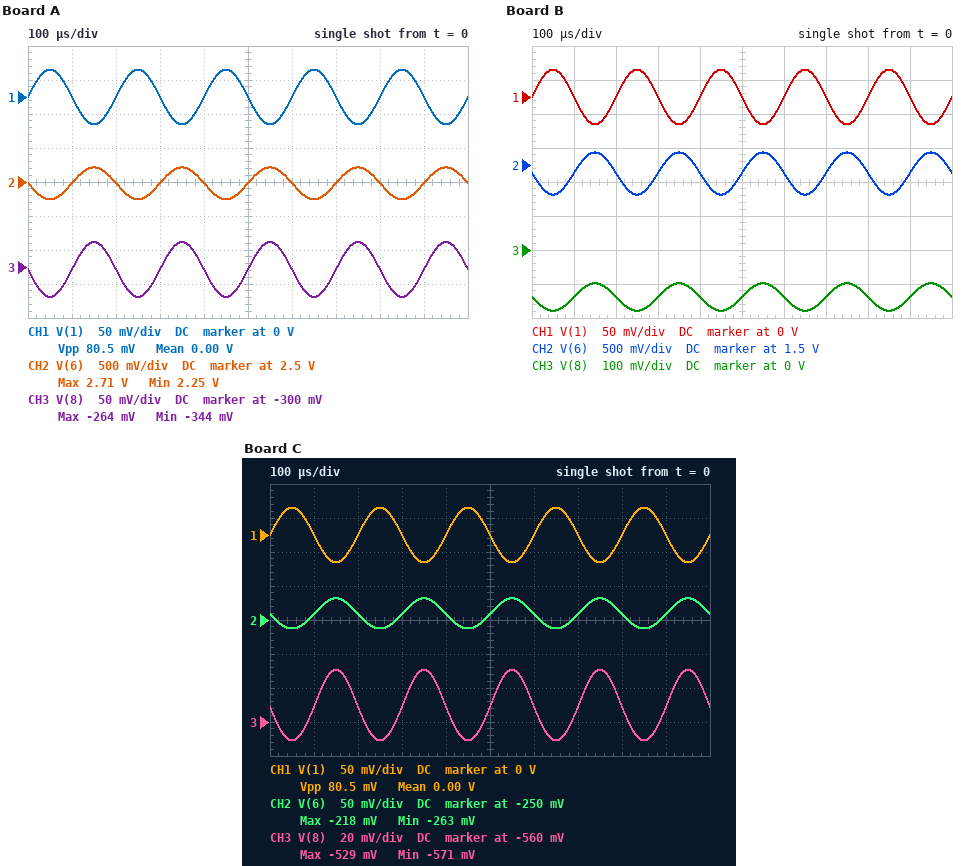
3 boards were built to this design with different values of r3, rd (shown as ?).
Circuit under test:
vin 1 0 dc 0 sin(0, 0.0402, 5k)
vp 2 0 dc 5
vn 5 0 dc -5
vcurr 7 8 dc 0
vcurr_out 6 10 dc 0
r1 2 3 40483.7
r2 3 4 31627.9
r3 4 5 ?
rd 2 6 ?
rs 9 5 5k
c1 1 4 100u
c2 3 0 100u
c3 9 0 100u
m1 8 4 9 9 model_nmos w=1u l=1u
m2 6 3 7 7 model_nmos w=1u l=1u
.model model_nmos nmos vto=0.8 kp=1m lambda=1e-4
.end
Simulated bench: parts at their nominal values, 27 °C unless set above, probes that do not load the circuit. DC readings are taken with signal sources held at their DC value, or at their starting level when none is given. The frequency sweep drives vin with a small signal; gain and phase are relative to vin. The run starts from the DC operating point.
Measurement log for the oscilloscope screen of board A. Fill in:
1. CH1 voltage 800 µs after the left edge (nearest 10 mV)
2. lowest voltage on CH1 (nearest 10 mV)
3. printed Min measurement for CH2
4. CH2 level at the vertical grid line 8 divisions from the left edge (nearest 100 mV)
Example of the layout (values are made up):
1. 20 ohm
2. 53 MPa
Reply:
1. 0 V
2. -40 mV
3. 2.25 V
4. 2.5 V
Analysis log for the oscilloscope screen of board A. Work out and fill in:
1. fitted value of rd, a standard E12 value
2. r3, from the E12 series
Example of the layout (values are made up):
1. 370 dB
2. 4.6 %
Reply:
1. 6.8 kΩ
2. 39 kΩ
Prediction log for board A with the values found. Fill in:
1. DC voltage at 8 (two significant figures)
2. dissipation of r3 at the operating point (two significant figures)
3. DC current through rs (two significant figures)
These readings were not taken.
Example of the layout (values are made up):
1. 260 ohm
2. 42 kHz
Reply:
1. -300 mV
2. 320 µW
3. 370 µA
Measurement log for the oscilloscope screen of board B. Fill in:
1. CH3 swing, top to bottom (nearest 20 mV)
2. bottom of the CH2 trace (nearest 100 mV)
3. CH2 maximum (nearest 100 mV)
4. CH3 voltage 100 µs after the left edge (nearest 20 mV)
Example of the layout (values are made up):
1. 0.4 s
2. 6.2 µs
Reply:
1. 80 mV
2. 1.1 V
3. 1.7 V
4. -140 mV
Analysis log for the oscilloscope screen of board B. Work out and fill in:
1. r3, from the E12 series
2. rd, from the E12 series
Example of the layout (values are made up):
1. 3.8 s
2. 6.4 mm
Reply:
1. 47 kΩ
2. 8.2 kΩ
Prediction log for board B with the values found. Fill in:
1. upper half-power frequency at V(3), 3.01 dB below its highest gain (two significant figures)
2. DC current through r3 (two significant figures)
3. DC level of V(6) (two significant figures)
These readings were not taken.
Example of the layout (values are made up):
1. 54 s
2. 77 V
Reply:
1. 200 mHz
2. 84 µA
3. 1.4 V
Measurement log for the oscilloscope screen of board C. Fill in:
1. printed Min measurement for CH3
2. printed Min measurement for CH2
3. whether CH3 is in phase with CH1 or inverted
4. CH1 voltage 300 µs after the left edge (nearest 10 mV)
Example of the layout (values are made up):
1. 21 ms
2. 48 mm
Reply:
1. -571 mV
2. -263 mV
3. inverted
4. 0 V
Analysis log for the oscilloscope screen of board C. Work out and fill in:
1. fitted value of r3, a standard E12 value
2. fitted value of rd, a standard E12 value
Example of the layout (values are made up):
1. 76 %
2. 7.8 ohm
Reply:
1. 120 kΩ
2. 6.8 kΩ
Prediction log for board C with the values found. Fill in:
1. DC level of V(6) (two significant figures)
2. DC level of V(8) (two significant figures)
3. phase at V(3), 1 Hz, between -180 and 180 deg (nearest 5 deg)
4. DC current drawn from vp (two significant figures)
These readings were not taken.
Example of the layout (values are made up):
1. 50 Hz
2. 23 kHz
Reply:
1. -240 mV
2. -550 mV
3. -80 deg
4. 820 µA
